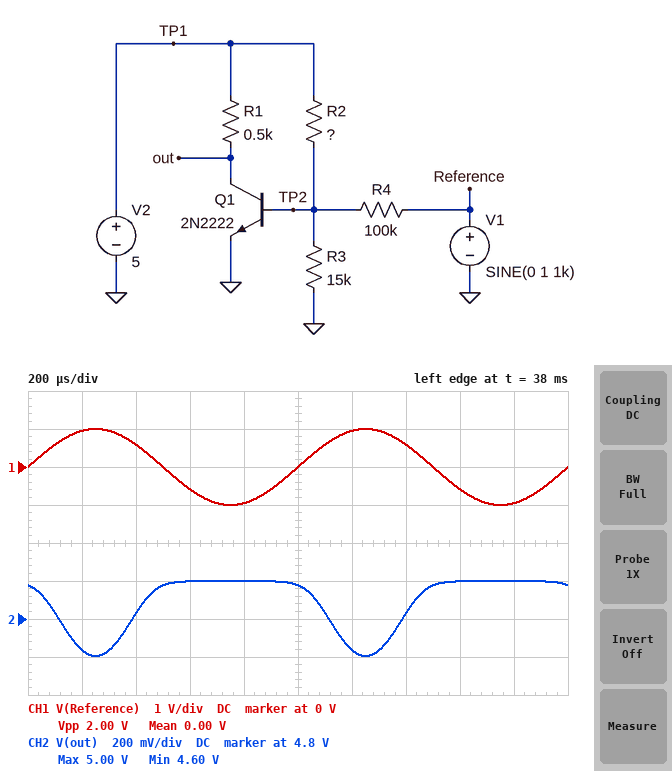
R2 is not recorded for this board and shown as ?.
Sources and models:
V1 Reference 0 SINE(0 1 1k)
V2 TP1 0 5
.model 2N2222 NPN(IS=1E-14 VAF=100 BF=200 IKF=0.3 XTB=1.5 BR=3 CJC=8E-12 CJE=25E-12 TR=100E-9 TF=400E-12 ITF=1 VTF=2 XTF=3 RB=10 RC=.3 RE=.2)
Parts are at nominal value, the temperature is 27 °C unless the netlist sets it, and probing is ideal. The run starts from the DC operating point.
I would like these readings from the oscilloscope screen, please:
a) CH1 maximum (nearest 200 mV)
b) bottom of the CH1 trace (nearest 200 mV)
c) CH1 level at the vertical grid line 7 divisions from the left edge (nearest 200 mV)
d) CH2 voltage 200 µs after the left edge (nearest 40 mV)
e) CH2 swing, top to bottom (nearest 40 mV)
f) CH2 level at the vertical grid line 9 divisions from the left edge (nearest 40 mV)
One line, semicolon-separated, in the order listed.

1.0 V; -1.0 V; 600 mV; 4.64 V; 400 mV; 5.00 V
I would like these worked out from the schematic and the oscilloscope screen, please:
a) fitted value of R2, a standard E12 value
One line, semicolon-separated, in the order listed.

100 kΩ
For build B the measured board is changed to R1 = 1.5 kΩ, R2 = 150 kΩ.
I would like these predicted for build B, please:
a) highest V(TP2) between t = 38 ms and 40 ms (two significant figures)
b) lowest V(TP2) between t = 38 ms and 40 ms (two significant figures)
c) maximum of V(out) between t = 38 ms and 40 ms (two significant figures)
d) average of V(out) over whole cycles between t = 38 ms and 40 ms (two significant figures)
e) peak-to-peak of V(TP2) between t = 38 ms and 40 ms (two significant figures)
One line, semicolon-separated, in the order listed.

520 mV; 280 mV; 5.0 V; 5.0 V; 240 mV
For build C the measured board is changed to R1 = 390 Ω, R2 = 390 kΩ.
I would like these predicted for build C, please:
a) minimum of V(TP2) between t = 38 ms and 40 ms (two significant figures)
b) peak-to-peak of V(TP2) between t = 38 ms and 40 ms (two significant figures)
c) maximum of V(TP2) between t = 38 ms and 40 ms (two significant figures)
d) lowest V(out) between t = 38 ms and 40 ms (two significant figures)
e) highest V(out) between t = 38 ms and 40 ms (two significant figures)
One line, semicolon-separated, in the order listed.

36 mV; 250 mV; 290 mV; 5.0 V; 5.0 V
